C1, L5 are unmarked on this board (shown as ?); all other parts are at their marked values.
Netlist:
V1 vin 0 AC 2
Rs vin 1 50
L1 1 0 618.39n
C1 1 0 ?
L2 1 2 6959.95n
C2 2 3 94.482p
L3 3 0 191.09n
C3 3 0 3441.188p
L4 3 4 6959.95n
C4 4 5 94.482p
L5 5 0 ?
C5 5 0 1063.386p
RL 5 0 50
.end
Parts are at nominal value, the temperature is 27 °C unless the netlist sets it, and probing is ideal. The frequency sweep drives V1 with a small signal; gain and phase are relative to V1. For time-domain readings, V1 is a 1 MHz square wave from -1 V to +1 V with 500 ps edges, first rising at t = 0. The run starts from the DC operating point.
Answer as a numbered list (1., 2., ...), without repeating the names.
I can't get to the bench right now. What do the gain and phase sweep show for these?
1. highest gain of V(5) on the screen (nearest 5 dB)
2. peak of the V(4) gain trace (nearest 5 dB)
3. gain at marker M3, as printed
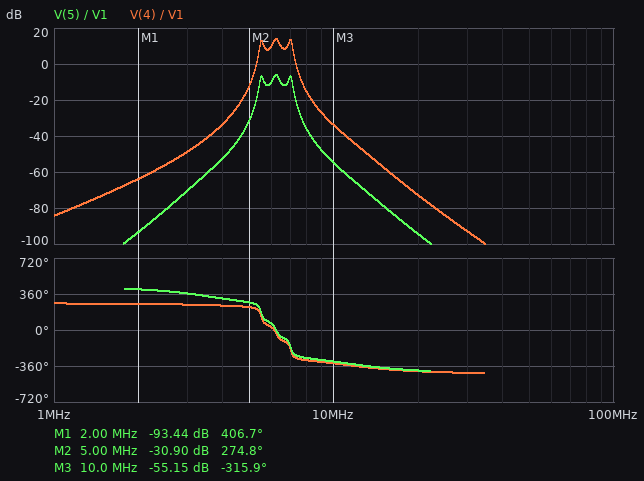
1. -5 dB
2. 15 dB
3. -55.15 dB
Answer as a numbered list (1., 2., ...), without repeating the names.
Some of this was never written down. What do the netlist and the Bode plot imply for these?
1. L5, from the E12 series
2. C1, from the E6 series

1. 1.8 µH
2. 330 pF
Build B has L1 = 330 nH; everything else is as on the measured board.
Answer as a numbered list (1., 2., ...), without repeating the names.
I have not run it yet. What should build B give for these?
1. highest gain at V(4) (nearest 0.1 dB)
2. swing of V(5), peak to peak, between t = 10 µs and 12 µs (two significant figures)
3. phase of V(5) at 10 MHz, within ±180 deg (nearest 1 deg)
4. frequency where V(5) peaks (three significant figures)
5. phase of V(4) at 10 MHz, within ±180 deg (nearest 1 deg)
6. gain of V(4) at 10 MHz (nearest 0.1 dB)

1. 12.9 dB
2. 130 mV
3. 78 deg
4. 5.54 MHz
5. 60 deg
6. -38.7 dB
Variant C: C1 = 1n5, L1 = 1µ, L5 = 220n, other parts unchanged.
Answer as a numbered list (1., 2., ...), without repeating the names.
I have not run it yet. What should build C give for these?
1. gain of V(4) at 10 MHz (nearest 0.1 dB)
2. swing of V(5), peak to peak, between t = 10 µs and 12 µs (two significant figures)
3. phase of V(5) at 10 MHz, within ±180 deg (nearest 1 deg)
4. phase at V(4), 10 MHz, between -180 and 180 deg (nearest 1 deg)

1. -47.2 dB
2. 140 mV
3. 40 deg
4. -49 deg
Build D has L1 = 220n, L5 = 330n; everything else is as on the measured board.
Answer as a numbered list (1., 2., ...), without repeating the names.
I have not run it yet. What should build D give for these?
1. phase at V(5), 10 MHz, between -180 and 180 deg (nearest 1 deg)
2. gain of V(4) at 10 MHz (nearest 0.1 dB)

1. 124 deg
2. -41.9 dB
